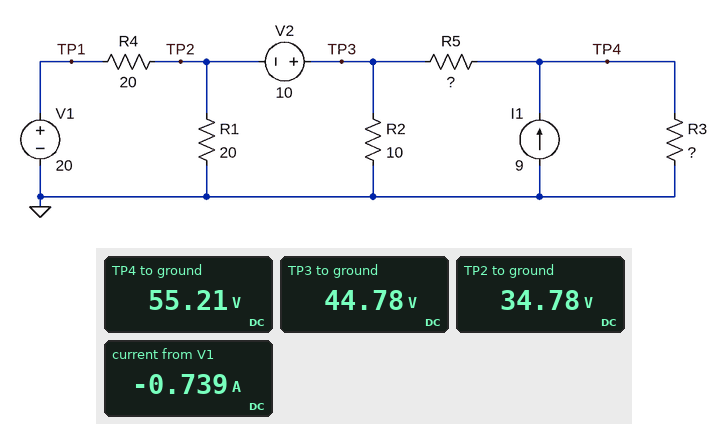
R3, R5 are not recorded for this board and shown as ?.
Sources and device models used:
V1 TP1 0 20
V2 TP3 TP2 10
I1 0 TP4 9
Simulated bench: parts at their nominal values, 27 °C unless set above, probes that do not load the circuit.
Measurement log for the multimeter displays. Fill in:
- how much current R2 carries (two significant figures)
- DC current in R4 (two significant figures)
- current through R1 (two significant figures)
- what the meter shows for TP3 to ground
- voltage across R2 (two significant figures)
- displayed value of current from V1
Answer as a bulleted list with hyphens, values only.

- 4.5 A
- 740 mA
- 1.7 A
- 44.78 V
- 45 V
- -0.739 A
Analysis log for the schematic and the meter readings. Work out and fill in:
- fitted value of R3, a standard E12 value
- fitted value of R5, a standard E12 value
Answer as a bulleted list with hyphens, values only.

- 27 Ω
- 1.5 Ω
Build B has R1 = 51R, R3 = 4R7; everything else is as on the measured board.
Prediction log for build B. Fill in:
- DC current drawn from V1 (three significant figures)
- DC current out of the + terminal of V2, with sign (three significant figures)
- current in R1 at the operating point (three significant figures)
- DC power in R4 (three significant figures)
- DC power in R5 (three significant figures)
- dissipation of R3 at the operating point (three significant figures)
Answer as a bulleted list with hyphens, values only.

- 213 mA
- -95.9 mA
- 309 mA
- 906 mW
- 10.7 W
- 188 W
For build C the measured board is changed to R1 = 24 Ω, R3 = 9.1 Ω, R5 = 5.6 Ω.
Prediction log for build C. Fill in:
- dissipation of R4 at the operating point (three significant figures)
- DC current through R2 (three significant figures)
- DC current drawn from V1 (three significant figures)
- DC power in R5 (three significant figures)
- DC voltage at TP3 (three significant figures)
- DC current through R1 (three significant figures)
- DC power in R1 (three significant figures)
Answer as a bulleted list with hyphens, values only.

- 67.9 mW
- 2.88 A
- 58.3 mA
- 73.0 W
- 28.8 V
- 785 mA
- 14.8 W
